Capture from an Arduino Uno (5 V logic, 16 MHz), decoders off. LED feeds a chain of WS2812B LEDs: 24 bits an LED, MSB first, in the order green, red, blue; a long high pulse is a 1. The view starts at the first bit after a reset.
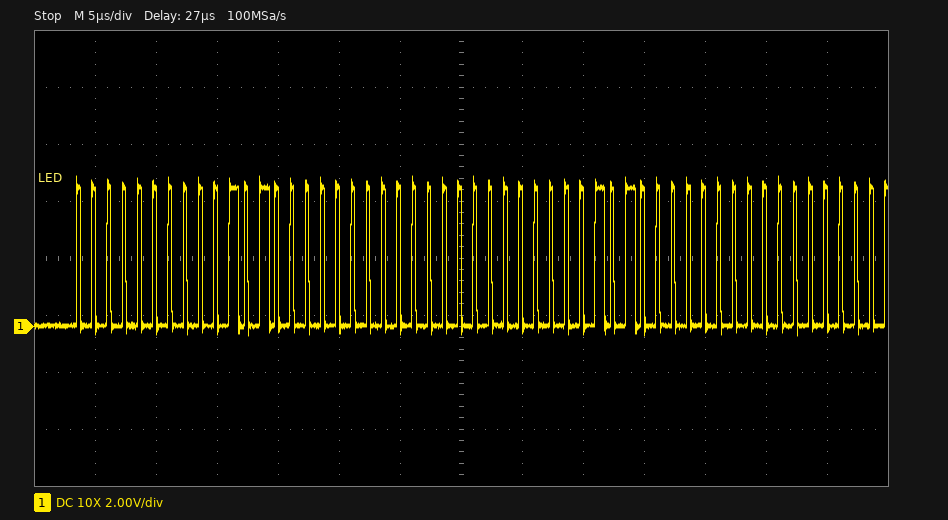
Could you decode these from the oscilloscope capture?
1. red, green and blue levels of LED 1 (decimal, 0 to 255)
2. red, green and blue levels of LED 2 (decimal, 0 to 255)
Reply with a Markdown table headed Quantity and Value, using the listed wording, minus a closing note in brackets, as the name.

| Quantity | Value |
|---|---|
| red, green and blue levels of LED 1 | 40, 0, 0 |
| red, green and blue levels of LED 2 | 40, 0, 0 |
